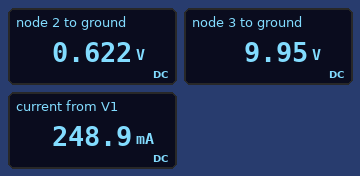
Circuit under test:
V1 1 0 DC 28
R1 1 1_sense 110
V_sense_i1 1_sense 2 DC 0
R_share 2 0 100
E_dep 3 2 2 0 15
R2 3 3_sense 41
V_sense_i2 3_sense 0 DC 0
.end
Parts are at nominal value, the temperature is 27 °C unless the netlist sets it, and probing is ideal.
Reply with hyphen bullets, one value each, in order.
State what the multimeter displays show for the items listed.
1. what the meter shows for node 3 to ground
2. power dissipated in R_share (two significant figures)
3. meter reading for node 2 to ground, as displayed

- 9.95 V
- 3.9 mW
- 0.622 V
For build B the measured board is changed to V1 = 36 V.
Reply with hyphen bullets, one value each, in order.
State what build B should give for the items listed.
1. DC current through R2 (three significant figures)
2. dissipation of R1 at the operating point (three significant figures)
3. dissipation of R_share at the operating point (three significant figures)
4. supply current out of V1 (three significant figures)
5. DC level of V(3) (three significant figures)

- 312 mA
- 11.3 W
- 6.39 mW
- 320 mA
- 12.8 V
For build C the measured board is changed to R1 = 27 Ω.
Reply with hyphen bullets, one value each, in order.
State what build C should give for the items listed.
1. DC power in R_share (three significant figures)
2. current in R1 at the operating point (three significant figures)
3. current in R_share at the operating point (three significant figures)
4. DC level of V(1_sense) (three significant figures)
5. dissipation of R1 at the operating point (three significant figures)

- 56.2 mW
- 949 mA
- 23.7 mA
- 2.37 V
- 24.3 W
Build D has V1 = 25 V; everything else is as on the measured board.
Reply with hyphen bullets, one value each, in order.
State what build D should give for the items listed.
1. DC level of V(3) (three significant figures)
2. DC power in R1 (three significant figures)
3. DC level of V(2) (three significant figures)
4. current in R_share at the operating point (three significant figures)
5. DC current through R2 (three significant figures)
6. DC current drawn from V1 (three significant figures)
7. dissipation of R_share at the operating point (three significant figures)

- 8.88 V
- 5.43 W
- 555 mV
- 5.55 mA
- 217 mA
- 222 mA
- 3.08 mW
